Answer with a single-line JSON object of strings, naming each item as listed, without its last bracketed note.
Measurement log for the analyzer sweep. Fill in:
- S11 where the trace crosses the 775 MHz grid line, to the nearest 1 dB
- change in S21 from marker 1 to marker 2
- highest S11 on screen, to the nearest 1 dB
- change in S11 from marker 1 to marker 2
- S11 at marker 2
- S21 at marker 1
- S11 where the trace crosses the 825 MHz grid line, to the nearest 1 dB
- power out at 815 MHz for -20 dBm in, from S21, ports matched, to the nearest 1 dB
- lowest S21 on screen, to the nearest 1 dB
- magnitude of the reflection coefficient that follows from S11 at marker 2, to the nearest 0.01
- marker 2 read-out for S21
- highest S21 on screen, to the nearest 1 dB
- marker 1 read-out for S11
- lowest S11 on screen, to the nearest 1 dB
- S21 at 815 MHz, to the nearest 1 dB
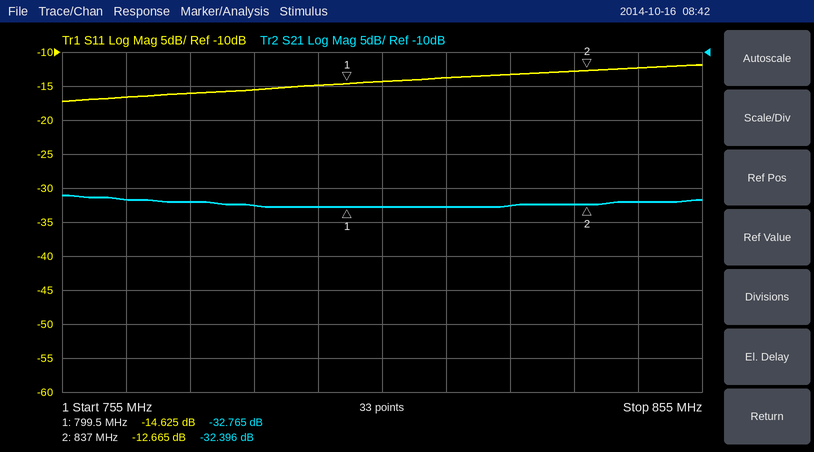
{"S11 where the trace crosses the 775 MHz grid line, to the nearest 1 dB": "-16 dB", "change in S21 from marker 1 to marker 2": "0.369 dB", "highest S11 on screen, to the nearest 1 dB": "-12 dB", "change in S11 from marker 1 to marker 2": "1.960 dB", "S11 at marker 2": "-12.665 dB", "S21 at marker 1": "-32.765 dB", "S11 where the trace crosses the 825 MHz grid line, to the nearest 1 dB": "-13 dB", "power out at 815 MHz for -20 dBm in, from S21, ports matched, to the nearest 1 dB": "-53 dBm", "lowest S21 on screen, to the nearest 1 dB": "-33 dB", "magnitude of the reflection coefficient that follows from S11 at marker 2, to the nearest 0.01": "0.23", "marker 2 read-out for S21": "-32.396 dB", "highest S21 on screen, to the nearest 1 dB": "-31 dB", "marker 1 read-out for S11": "-14.625 dB", "lowest S11 on screen, to the nearest 1 dB": "-17 dB", "S21 at 815 MHz, to the nearest 1 dB": "-33 dB"}
